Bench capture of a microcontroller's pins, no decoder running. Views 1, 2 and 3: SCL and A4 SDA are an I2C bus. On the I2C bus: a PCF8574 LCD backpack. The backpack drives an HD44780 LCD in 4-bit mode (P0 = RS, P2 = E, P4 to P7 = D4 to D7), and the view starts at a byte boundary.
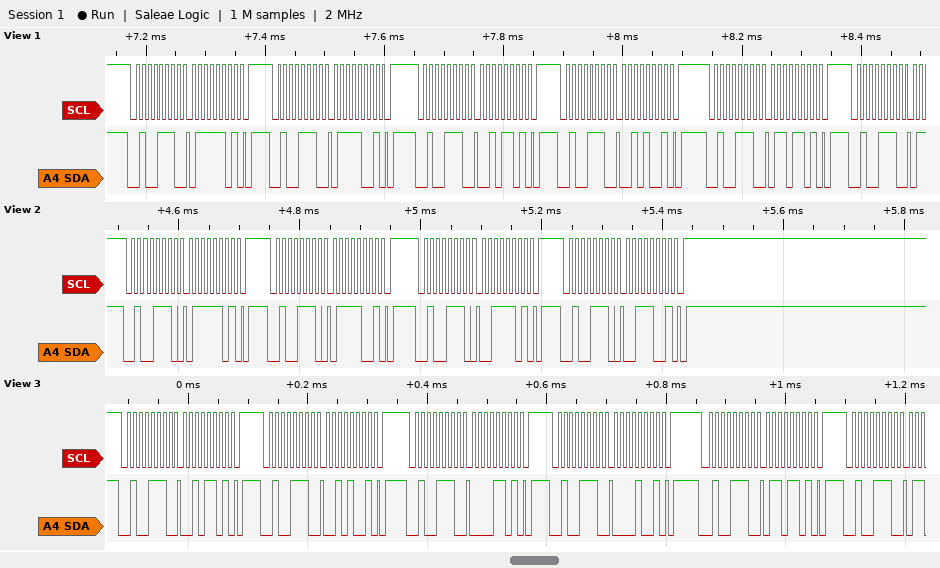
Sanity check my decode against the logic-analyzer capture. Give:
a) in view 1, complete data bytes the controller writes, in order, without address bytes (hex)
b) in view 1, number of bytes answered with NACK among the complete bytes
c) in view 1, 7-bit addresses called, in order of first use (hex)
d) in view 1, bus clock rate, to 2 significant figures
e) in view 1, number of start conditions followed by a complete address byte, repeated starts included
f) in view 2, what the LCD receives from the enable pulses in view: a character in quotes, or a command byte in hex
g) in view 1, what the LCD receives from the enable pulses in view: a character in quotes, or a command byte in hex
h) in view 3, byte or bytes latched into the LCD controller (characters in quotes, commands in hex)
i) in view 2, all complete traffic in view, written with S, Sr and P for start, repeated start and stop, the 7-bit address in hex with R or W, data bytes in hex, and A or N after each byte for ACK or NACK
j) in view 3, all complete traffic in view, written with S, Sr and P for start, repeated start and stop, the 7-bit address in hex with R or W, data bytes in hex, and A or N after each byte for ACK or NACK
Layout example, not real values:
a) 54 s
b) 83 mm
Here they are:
a) 7D 79 2D 29 6D
b) 0
c) 0x27
d) 100 kHz
e) 6
f) 's'
g) 'r'
h) ' '
i) S 27W A 7D A P S 27W A 79 A P S 27W A 3D A P S 27W A 39 A P
j) S 27W A 2D A P S 27W A 29 A P S 27W A 0D A P S 27W A 09 A P S 27W A 6D A P S 27W A
